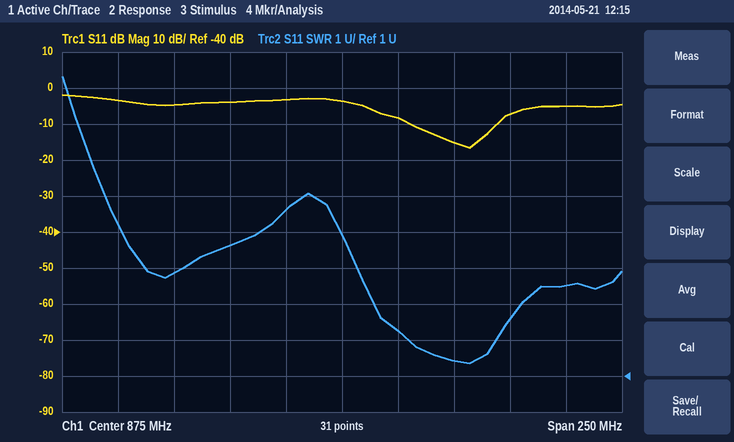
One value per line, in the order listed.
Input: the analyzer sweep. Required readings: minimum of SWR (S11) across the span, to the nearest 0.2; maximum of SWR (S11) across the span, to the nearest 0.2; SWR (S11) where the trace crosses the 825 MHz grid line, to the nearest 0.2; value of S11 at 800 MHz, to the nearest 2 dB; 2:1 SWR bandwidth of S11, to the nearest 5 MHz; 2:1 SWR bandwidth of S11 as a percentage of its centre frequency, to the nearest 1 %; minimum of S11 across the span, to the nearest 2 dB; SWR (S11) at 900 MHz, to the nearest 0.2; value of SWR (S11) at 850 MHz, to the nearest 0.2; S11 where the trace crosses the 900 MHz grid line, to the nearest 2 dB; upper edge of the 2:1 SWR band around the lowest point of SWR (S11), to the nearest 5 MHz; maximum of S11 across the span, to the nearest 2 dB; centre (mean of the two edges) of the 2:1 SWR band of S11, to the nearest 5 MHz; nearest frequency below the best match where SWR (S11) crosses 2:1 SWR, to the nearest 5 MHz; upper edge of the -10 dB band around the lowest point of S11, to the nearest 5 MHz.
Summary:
1.4
9.4
4.6
-4 dB
40 MHz
4 %
-16 dB
2.2
5.6
-8 dB
945 MHz
-2 dB
925 MHz
905 MHz
945 MHz
